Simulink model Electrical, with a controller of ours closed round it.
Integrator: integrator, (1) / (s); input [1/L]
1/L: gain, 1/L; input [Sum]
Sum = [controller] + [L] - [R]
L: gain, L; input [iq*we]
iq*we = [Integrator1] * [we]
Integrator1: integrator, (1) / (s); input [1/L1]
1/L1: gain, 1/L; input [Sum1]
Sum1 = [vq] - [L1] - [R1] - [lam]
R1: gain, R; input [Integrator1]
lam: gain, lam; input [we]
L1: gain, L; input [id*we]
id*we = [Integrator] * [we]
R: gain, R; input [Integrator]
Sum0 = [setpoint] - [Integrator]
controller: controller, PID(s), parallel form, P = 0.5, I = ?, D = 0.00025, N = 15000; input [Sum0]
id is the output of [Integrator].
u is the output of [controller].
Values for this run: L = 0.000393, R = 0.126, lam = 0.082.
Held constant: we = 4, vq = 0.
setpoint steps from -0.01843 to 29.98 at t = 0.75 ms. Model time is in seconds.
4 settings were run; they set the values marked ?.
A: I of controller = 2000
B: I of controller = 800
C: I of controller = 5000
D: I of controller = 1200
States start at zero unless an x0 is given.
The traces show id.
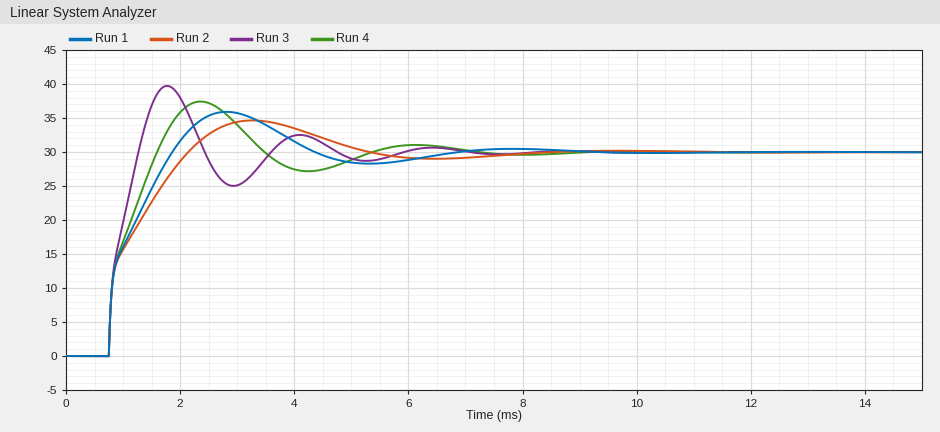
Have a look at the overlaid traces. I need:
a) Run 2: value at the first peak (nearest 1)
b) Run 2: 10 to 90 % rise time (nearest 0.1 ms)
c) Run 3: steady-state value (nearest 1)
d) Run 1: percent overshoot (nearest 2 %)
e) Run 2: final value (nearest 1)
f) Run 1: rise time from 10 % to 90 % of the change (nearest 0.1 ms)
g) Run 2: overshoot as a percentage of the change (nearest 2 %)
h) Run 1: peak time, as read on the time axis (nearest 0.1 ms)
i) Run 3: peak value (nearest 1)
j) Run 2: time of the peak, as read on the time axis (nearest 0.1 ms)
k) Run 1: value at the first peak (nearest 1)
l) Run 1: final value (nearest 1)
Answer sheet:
35
1.1 ms
30
20 %
30
0.9 ms
16 %
2.8 ms
40
3.3 ms
36
30
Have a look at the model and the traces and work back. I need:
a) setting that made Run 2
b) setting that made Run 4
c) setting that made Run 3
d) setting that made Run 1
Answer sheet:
B
A
C
D
